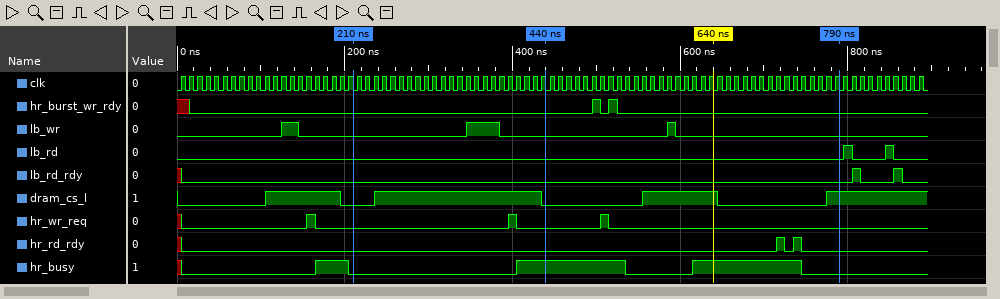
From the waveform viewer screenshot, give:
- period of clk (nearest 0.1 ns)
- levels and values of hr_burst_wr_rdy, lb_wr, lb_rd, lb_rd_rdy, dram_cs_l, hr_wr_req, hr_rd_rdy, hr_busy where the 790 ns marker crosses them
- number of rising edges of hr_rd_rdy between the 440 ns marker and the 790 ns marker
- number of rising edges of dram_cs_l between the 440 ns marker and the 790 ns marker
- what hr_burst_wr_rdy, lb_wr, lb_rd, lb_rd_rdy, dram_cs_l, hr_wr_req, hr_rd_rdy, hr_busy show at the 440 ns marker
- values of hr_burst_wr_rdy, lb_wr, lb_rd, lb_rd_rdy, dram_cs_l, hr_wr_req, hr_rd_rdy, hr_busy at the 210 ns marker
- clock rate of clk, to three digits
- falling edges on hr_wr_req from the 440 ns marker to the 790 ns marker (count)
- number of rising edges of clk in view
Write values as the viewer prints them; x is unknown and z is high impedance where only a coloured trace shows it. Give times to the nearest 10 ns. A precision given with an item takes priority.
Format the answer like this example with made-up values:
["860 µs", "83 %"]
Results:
["10 ns", "hr_burst_wr_rdy=0, lb_wr=0, lb_rd=0, lb_rd_rdy=0, dram_cs_l=1, hr_wr_req=0, hr_rd_rdy=0, hr_busy=0", "2", "2", "hr_burst_wr_rdy=0, lb_wr=0, lb_rd=0, lb_rd_rdy=0, dram_cs_l=0, hr_wr_req=0, hr_rd_rdy=0, hr_busy=1", "hr_burst_wr_rdy=0, lb_wr=0, lb_rd=0, lb_rd_rdy=0, dram_cs_l=0, hr_wr_req=0, hr_rd_rdy=0, hr_busy=0", "100 MHz", "1", "89"]
